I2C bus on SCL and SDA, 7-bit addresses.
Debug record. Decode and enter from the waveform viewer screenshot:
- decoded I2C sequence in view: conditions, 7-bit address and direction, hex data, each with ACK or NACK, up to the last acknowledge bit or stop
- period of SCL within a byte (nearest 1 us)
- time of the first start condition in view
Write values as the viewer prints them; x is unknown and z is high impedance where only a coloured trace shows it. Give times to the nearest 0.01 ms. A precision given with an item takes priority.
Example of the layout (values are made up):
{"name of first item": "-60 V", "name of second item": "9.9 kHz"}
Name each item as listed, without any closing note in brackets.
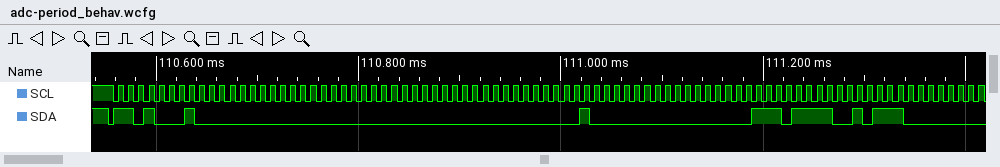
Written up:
{"decoded I2C sequence in view: conditions, 7-bit address and direction, hex data, each with ACK or NACK, up to the last acknowledge bit or stop": "start, address 68 read ACK, 00 ACK, 00 ACK, 00 ACK, 00 ACK, 40 ACK, 00 ACK, EF ACK, 5C ACK", "period of SCL within a byte": "10 us", "time of the first start condition in view": "110.55 ms"}
